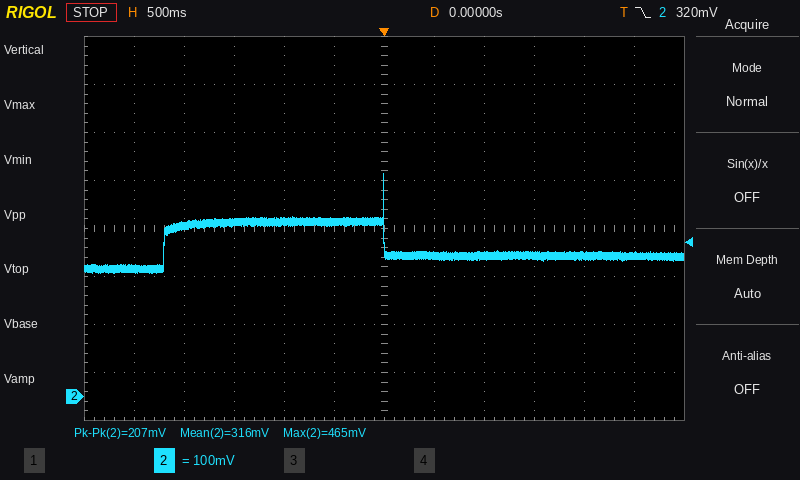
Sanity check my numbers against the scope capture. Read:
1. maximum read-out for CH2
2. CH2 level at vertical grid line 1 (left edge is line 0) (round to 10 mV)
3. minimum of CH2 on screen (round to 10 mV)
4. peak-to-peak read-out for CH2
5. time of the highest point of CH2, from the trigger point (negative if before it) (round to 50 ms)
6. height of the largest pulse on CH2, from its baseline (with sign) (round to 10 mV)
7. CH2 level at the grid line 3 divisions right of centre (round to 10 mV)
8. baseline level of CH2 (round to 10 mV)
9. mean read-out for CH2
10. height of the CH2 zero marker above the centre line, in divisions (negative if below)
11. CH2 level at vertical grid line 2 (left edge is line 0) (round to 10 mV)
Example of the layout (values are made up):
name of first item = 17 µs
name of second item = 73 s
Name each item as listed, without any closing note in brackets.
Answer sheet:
maximum read-out for CH2 = 465 mV
CH2 level at vertical grid line 1 (left edge is line 0) = 270 mV
minimum of CH2 on screen = 260 mV
peak-to-peak read-out for CH2 = 207 mV
time of the highest point of CH2, from the trigger point (negative if before it) = 0 ms
height of the largest pulse on CH2, from its baseline (with sign) = +170 mV
CH2 level at the grid line 3 divisions right of centre = 290 mV
baseline level of CH2 = 290 mV
mean read-out for CH2 = 316 mV
height of the CH2 zero marker above the centre line, in divisions = -3.5 div
CH2 level at vertical grid line 2 (left edge is line 0) = 360 mV
